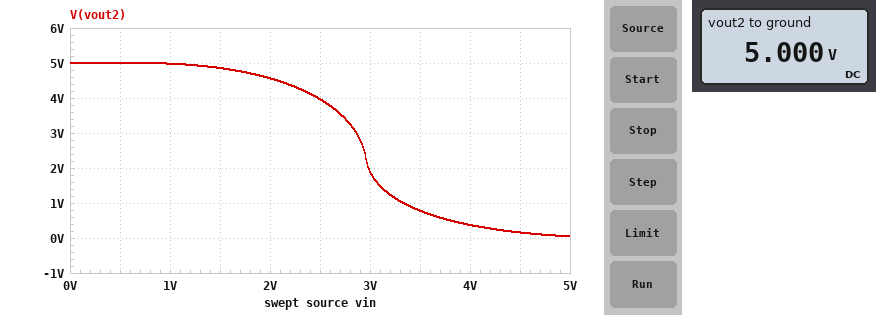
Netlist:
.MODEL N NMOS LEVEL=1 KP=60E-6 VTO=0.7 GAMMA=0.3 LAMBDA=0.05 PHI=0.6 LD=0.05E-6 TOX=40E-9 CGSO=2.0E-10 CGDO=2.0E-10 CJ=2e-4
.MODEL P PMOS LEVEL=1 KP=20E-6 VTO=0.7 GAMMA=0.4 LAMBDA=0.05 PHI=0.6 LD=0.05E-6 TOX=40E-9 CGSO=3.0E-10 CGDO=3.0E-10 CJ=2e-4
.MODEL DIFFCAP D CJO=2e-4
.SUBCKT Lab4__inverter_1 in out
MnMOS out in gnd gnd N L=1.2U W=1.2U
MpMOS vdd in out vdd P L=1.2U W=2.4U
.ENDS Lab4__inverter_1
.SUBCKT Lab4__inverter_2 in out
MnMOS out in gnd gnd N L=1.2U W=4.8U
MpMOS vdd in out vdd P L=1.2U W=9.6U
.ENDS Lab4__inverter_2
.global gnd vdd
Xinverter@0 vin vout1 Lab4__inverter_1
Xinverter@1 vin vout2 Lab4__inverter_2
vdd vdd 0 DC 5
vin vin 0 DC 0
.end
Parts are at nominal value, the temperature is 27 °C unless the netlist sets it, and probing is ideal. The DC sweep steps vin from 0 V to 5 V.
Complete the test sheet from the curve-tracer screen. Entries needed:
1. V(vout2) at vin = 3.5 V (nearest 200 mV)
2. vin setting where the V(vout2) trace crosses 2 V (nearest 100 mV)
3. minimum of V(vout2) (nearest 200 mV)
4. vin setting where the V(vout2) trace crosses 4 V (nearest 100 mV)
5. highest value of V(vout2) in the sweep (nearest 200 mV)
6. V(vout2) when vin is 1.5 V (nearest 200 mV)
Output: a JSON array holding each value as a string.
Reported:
["800 mV", "3.0 V", "0 V", "2.5 V", "5.0 V", "4.8 V"]
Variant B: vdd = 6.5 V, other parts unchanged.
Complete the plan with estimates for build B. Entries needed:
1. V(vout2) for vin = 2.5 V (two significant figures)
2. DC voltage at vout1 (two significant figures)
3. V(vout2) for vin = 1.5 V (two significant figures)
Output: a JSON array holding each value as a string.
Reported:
["5.8 V", "6.5 V", "6.4 V"]
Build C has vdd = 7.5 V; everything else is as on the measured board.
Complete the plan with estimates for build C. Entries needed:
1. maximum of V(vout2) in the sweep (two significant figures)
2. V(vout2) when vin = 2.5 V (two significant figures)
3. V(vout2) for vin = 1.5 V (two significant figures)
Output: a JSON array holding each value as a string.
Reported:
["7.5 V", "6.9 V", "7.4 V"]
